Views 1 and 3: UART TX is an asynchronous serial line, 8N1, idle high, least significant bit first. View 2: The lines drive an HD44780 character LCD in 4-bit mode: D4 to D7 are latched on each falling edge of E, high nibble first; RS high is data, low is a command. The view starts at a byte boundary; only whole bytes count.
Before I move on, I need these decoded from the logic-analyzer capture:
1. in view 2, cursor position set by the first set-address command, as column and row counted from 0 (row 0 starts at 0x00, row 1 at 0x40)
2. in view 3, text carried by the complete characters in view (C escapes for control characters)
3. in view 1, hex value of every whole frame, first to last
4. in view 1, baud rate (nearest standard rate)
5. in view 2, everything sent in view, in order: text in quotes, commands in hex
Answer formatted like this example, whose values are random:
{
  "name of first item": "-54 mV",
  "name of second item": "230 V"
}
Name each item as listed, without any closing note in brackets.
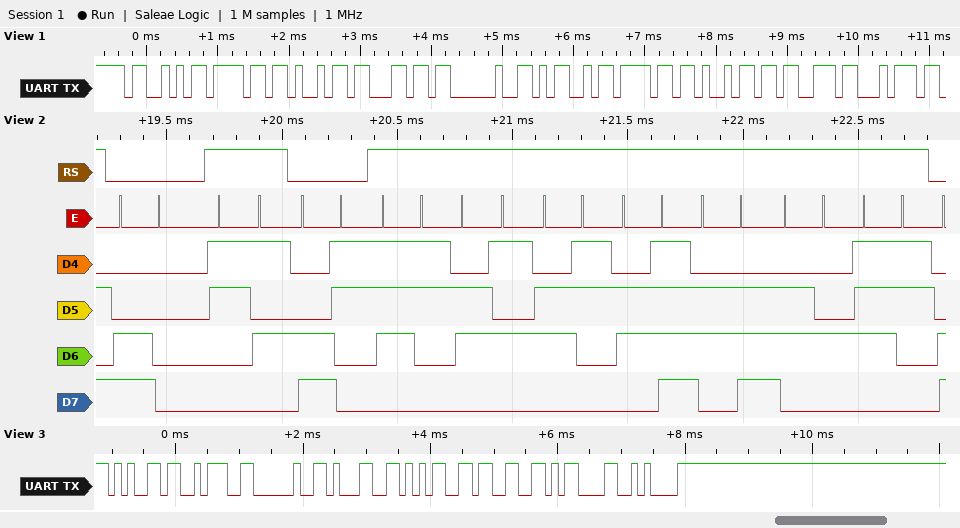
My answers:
{
  "in view 2, cursor position set by the first set-address command, as column and row counted from 0": "column 0, row 1",
  "in view 3, text carried by the complete characters in view": "\"e: 153\\r\\n\"",
  "in view 1, hex value of every whole frame, first to last": "53 6F 69 6C 20 4D 6F 69 73 74",
  "in view 1, baud rate": "9600 baud",
  "in view 2, everything sent in view, in order: text in quotes, commands in hex": "0xC0 \"5\" 0xC3 \"seconds\""
}
